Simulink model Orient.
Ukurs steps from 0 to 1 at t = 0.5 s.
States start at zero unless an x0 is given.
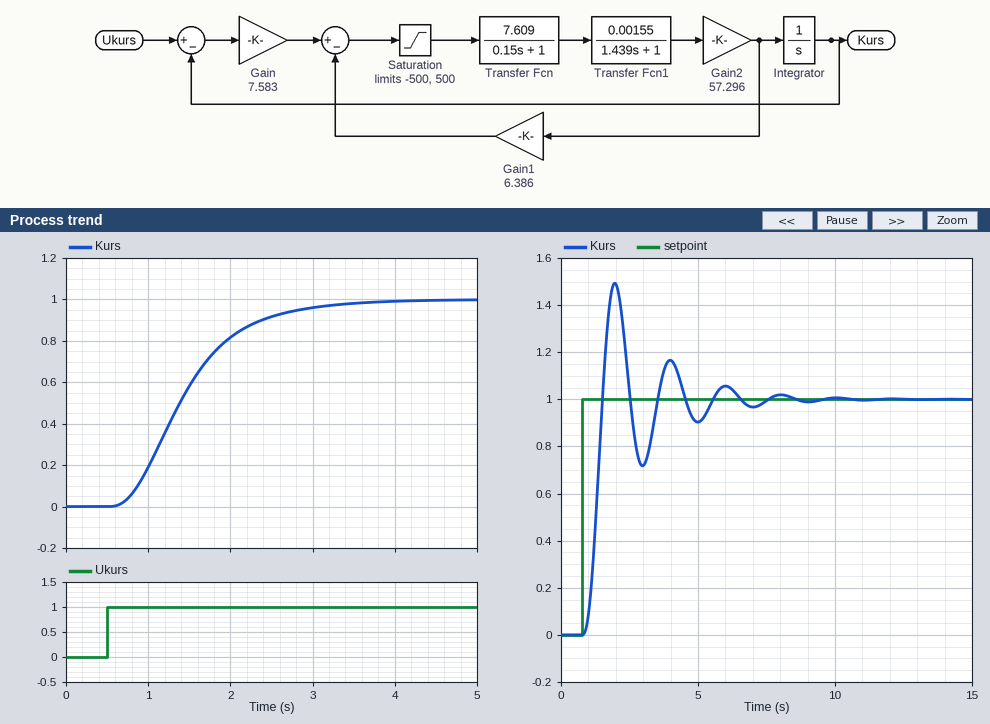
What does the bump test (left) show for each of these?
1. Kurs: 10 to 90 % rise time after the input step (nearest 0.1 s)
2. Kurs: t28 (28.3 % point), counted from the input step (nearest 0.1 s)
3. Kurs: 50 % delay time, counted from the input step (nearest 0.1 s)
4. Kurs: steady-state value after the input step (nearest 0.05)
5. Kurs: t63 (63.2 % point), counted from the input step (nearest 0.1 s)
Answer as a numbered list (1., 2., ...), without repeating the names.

1. 1.5 s
2. 0.6 s
3. 0.9 s
4. 1.00
5. 1.1 s
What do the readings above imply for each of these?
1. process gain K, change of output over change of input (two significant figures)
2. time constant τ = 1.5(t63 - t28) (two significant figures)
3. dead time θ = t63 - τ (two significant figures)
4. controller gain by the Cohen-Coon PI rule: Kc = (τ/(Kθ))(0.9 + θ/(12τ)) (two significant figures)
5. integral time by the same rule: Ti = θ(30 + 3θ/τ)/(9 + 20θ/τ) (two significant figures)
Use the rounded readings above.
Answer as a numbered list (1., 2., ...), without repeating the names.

1. 1.0
2. 0.75 s
3. 0.35 s
4. 2.0
5. 0.60 s
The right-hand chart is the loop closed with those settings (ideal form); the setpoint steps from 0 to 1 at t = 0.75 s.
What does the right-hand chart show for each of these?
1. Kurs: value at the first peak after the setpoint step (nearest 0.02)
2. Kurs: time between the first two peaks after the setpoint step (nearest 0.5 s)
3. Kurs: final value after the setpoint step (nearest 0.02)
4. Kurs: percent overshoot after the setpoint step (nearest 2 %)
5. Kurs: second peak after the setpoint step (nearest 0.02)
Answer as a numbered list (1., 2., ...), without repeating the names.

1. 1.50
2. 2.0 s
3. 1.00
4. 50 %
5. 1.16
